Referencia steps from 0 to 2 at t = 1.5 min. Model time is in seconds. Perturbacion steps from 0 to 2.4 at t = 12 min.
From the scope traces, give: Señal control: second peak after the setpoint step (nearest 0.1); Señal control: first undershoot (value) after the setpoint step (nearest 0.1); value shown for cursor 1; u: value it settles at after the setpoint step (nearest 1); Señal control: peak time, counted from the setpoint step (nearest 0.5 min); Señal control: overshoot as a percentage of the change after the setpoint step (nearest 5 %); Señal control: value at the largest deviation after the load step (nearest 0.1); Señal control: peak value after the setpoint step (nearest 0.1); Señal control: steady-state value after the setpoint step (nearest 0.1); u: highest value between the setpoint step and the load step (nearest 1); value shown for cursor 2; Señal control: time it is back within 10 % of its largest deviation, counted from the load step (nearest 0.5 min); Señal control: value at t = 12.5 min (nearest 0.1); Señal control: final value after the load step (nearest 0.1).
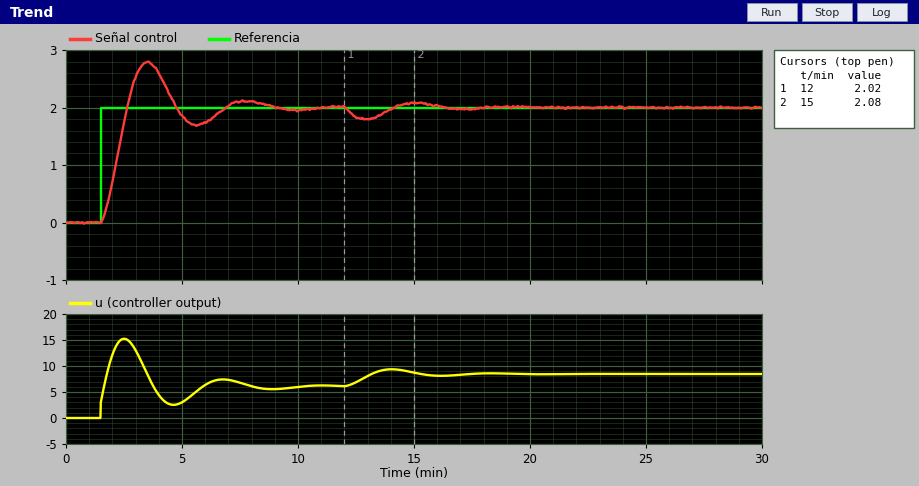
2.1
1.7
2.02
6
2.0 min
40 %
1.8
2.8
2.0
15
2.08
5.5 min
1.8
2.0
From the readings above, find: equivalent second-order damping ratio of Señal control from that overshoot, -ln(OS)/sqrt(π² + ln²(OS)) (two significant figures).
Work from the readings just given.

0.28
